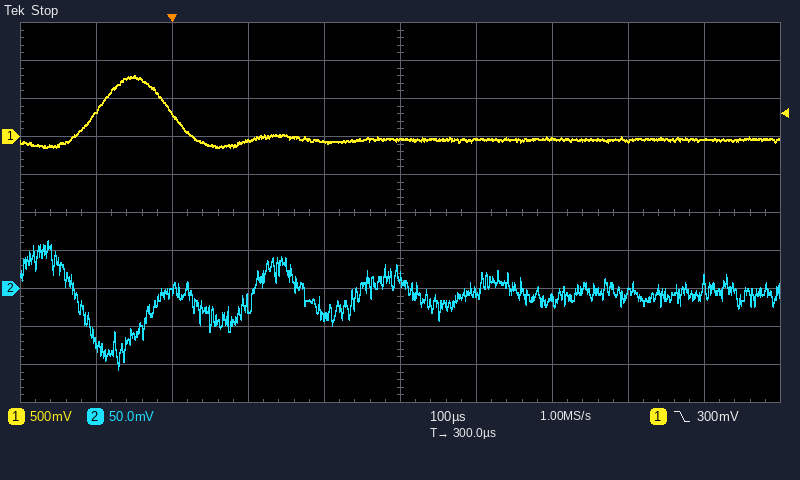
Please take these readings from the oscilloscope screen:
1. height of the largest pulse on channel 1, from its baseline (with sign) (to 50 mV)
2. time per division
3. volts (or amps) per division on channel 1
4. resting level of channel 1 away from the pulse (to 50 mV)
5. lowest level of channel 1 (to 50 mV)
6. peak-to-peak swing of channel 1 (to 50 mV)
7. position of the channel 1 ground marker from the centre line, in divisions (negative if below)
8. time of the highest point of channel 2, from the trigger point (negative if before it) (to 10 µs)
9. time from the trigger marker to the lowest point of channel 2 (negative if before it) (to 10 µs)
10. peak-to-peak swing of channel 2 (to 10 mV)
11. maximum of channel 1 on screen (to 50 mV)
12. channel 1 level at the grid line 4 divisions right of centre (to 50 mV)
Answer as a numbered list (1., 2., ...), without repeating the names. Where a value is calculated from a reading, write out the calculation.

1. 800 mV − (-50 mV) = +850 mV
2. 100 µs
3. 500 mV
4. -50 mV
5. -150 mV
6. 800 mV − (-150 mV) = 950 mV
7. +2.0 div
8. -160 µs
9. -70 µs
10. 170 mV
11. 800 mV
12. -50 mV
